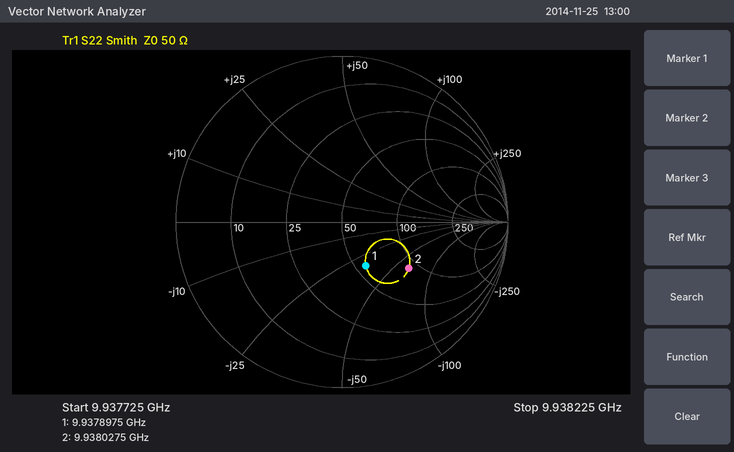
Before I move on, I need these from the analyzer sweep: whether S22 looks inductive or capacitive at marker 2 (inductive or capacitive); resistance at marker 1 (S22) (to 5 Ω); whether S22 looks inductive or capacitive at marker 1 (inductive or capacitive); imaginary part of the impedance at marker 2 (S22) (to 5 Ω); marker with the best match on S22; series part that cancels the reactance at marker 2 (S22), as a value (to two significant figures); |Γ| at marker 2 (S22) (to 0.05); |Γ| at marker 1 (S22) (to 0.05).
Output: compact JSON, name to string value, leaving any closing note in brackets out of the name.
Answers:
{"whether S22 looks inductive or capacitive at marker 2": "capacitive", "resistance at marker 1 (S22)": "55 Ω", "whether S22 looks inductive or capacitive at marker 1": "capacitive", "imaginary part of the impedance at marker 2 (S22)": "-65 Ω", "marker with the best match on S22": "marker 1", "series part that cancels the reactance at marker 2 (S22), as a value": "1.0 nH", "|Γ| at marker 2 (S22)": "0.50", "|Γ| at marker 1 (S22)": "0.30"}
